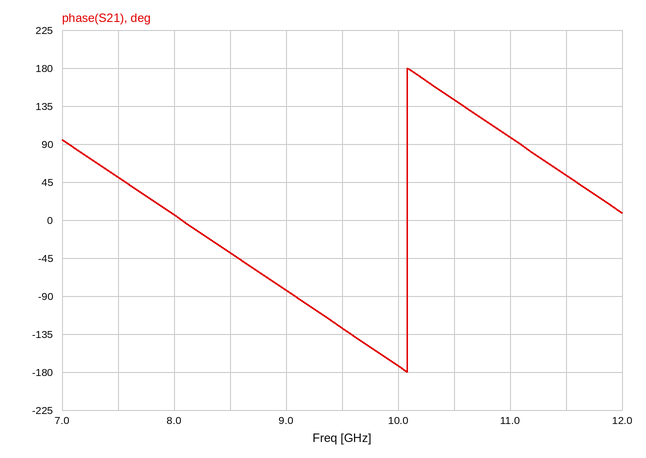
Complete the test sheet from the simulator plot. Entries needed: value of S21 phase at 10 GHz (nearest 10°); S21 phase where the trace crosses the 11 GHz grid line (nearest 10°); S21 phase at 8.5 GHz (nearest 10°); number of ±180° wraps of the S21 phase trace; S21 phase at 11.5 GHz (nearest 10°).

-170°
100°
-40°
1
50°
